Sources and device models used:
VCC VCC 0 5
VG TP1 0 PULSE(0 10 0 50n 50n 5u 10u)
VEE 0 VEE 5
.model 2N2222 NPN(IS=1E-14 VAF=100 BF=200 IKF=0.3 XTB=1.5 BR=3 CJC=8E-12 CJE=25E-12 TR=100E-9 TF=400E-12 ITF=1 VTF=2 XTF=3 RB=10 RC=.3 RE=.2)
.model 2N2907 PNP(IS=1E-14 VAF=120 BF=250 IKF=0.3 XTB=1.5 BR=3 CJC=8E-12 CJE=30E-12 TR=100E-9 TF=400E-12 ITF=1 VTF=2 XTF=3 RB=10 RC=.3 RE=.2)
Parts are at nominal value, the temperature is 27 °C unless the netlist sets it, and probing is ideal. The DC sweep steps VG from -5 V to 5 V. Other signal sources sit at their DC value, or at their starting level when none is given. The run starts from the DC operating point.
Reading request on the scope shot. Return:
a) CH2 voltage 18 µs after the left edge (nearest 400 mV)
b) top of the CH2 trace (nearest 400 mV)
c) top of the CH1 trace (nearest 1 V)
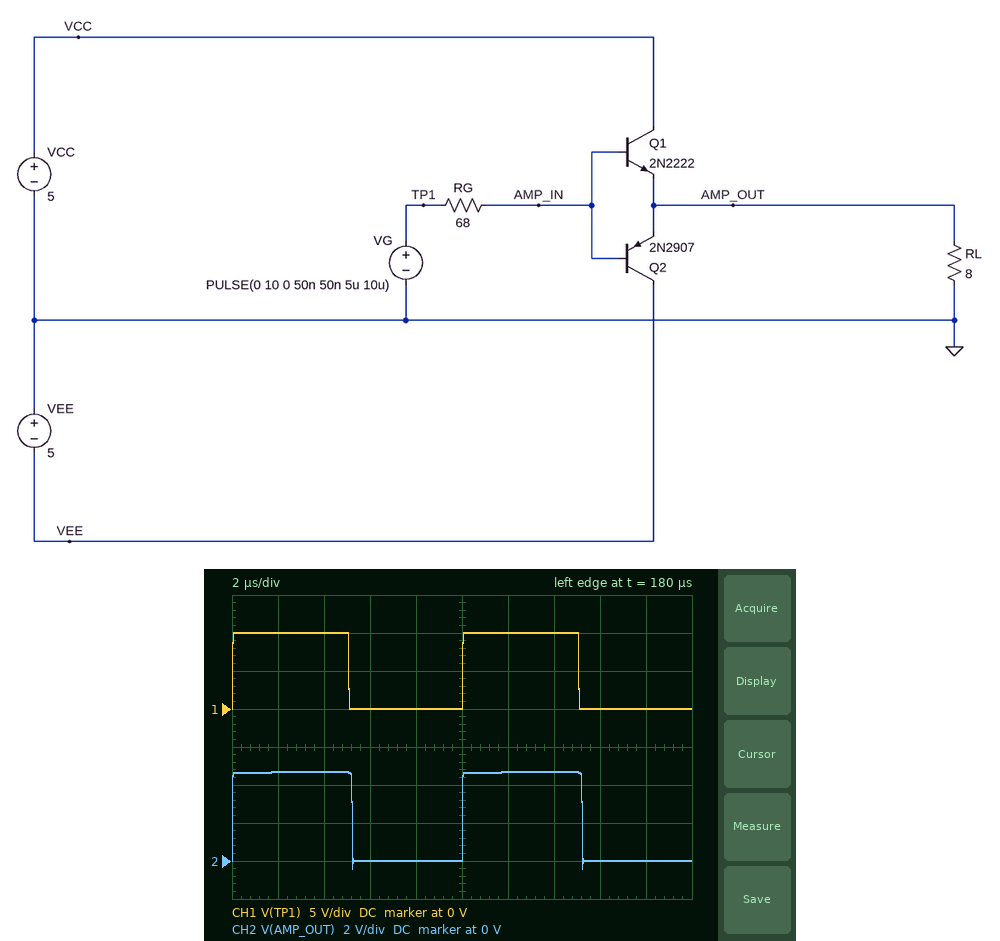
0 V
4.8 V
10 V
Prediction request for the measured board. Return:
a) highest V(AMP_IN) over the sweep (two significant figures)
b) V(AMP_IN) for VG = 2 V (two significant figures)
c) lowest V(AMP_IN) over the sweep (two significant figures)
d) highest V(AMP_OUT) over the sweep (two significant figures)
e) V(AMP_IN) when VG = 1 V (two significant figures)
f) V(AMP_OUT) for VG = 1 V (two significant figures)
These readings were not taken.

4.6 V
1.9 V
-4.7 V
3.6 V
990 mV
240 mV
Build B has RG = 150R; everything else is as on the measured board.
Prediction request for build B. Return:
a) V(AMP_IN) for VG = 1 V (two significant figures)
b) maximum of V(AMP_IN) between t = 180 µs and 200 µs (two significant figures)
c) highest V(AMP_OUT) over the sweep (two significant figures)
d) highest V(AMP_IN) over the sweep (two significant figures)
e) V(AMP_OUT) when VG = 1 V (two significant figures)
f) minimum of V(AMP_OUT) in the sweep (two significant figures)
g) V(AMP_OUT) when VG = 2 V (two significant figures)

980 mV
5.9 V
3.3 V
4.3 V
230 mV
-3.4 V
1.0 V
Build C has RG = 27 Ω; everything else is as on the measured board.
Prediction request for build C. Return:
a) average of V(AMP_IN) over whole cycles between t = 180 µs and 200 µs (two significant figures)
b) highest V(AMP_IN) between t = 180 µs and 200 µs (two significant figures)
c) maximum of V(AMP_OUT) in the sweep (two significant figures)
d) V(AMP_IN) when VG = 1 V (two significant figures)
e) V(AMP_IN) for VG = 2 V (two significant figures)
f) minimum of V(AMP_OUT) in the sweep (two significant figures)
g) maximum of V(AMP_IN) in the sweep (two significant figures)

3.5 V
6.8 V
3.8 V
1.0 V
2.0 V
-3.9 V
4.8 V
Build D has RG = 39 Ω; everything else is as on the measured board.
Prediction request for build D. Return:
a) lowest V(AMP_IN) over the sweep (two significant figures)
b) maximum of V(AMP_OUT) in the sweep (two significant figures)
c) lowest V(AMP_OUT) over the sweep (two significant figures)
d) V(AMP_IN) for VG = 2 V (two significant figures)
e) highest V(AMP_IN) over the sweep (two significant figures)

-4.8 V
3.8 V
-3.8 V
2.0 V
4.8 V
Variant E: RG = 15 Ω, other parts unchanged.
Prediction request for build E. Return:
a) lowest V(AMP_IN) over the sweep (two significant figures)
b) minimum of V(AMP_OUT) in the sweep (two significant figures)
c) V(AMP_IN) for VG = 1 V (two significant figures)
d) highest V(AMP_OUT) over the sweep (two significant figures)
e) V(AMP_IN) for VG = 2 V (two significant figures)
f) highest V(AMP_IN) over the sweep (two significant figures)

-4.9 V
-3.9 V
1.0 V
3.9 V
2.0 V
4.9 V
